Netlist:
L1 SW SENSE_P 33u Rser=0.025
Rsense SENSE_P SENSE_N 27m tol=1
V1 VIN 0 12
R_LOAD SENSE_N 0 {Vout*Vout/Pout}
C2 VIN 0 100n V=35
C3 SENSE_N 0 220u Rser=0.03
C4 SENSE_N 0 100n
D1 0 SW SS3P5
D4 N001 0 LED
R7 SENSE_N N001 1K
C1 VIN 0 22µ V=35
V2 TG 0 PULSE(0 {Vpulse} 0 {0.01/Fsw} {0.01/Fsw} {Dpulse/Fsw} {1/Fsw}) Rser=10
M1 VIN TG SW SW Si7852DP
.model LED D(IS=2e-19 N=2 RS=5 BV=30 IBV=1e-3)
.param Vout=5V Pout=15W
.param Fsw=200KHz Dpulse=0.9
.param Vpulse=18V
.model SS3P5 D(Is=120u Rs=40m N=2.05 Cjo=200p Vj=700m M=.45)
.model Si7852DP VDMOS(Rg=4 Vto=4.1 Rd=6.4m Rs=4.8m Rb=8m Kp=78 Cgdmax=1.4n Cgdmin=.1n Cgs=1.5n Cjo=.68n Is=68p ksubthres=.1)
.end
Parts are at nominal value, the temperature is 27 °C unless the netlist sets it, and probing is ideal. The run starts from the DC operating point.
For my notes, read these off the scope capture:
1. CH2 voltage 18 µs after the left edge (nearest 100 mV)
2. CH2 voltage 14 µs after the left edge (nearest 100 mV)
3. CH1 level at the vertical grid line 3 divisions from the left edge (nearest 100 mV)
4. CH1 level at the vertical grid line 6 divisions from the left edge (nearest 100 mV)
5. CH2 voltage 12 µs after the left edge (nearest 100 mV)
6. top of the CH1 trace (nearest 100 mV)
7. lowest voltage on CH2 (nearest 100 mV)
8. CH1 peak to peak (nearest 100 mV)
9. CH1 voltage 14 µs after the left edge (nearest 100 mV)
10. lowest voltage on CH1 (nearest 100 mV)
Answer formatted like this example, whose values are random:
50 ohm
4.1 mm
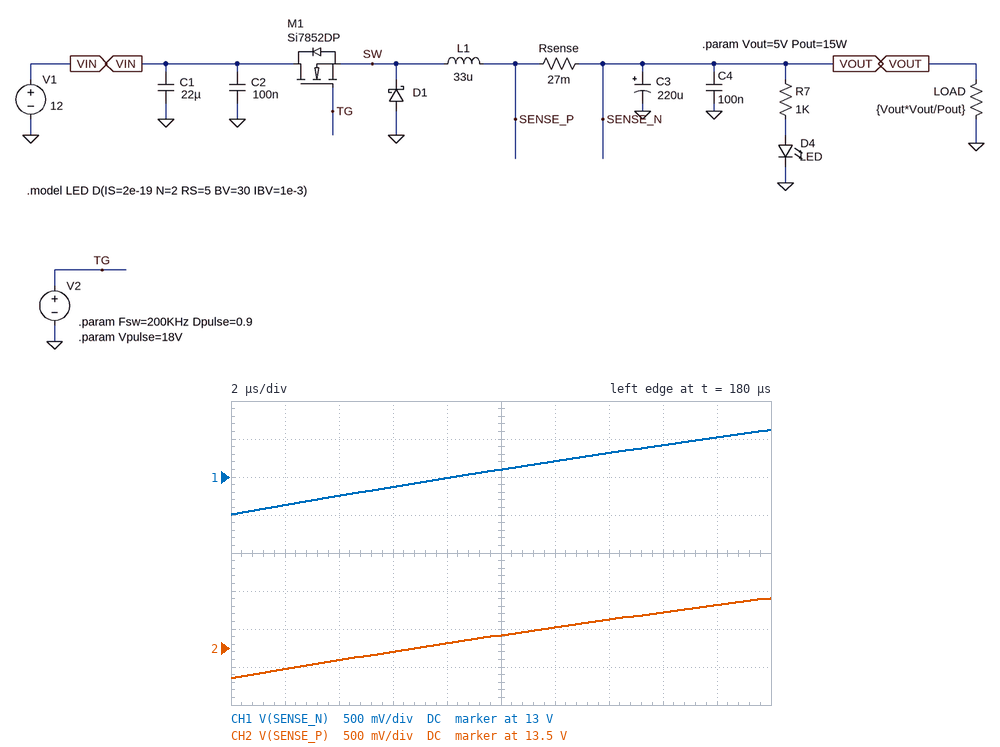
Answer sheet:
14.1 V
13.9 V
12.9 V
13.2 V
13.8 V
13.6 V
13.1 V
1.1 V
13.3 V
12.5 V
